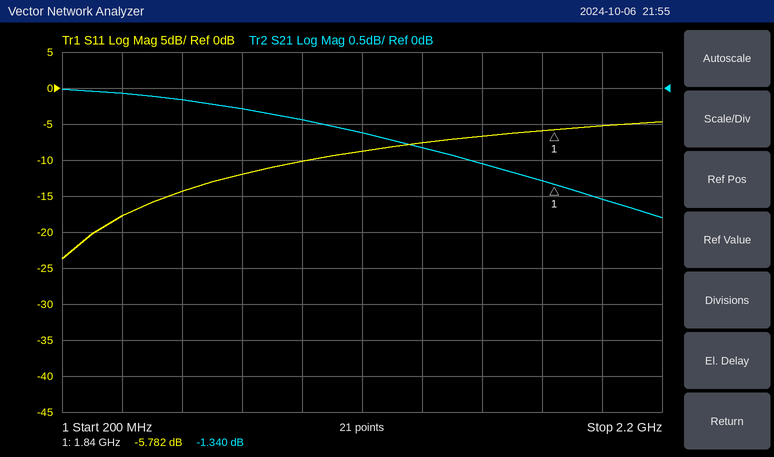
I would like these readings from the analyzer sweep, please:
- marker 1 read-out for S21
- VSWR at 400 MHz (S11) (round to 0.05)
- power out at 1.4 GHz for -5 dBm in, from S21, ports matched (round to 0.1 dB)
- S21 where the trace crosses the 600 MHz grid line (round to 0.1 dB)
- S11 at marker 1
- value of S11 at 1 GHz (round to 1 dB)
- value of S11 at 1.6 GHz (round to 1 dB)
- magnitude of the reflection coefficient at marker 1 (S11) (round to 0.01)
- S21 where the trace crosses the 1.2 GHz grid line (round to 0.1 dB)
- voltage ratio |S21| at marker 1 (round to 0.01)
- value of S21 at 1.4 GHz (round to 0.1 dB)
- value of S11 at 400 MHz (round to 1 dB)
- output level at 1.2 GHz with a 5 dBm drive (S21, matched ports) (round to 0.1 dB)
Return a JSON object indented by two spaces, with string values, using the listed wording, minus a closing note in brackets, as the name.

{
  "marker 1 read-out for S21": "-1.340 dB",
  "VSWR at 400 MHz (S11)": "1.30",
  "power out at 1.4 GHz for -5 dBm in, from S21, ports matched": "-5.8 dBm",
  "S21 where the trace crosses the 600 MHz grid line": "-0.2 dB",
  "S11 at marker 1": "-5.782 dB",
  "value of S11 at 1 GHz": "-10 dB",
  "value of S11 at 1.6 GHz": "-7 dB",
  "magnitude of the reflection coefficient at marker 1 (S11)": "0.51",
  "S21 where the trace crosses the 1.2 GHz grid line": "-0.6 dB",
  "voltage ratio |S21| at marker 1": "0.86",
  "value of S21 at 1.4 GHz": "-0.8 dB",
  "value of S11 at 400 MHz": "-18 dB",
  "output level at 1.2 GHz with a 5 dBm drive (S21, matched ports)": "4.4 dBm"
}
